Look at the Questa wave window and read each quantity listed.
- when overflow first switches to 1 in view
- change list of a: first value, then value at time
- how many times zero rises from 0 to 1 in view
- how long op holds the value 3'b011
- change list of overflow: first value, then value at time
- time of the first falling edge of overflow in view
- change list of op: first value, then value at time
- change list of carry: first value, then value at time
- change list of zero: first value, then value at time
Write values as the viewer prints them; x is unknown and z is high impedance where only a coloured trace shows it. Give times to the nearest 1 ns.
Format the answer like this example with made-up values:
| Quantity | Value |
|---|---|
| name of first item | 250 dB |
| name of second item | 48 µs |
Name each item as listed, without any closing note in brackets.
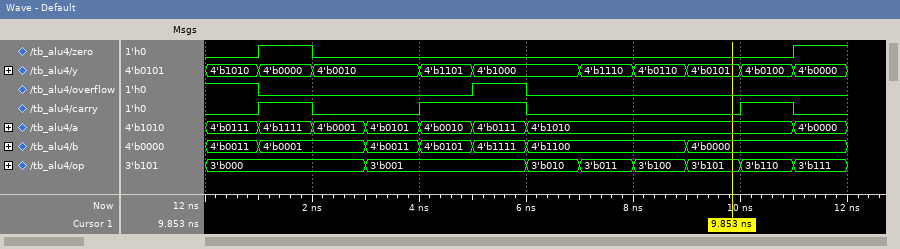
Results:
| Quantity | Value |
|---|---|
| when overflow first switches to 1 in view | 5 ns |
| change list of a: first value, then value at time | 4'b0111, 4'b1111 at 1 ns, 4'b0001 at 2 ns, 4'b0101 at 3 ns, 4'b0010 at 4 ns, 4'b0111 at 5 ns, 4'b1010 at 6 ns, 4'b0000 at 11 ns |
| how many times zero rises from 0 to 1 in view | 2 |
| how long op holds the value 3'b011 | 1 ns |
| change list of overflow: first value, then value at time | 1, 0 at 1 ns, 1 at 5 ns, 0 at 6 ns |
| time of the first falling edge of overflow in view | 1 ns |
| change list of op: first value, then value at time | 3'b000, 3'b001 at 3 ns, 3'b010 at 6 ns, 3'b011 at 7 ns, 3'b100 at 8 ns, 3'b101 at 9 ns, 3'b110 at 10 ns, 3'b111 at 11 ns |
| change list of carry: first value, then value at time | 0, 1 at 1 ns, 0 at 2 ns, 1 at 4 ns, 0 at 6 ns, 1 at 10 ns, 0 at 11 ns |
| change list of zero: first value, then value at time | 0, 1 at 1 ns, 0 at 2 ns, 1 at 11 ns |
